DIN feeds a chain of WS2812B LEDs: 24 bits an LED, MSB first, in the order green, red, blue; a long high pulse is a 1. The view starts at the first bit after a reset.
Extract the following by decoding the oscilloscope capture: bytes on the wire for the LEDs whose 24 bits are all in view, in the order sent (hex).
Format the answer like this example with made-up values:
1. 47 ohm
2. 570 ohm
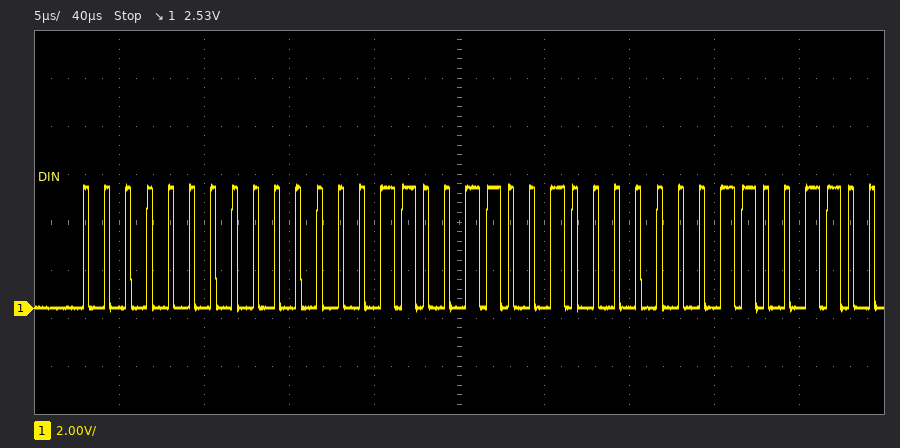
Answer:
1. 00 03 32
